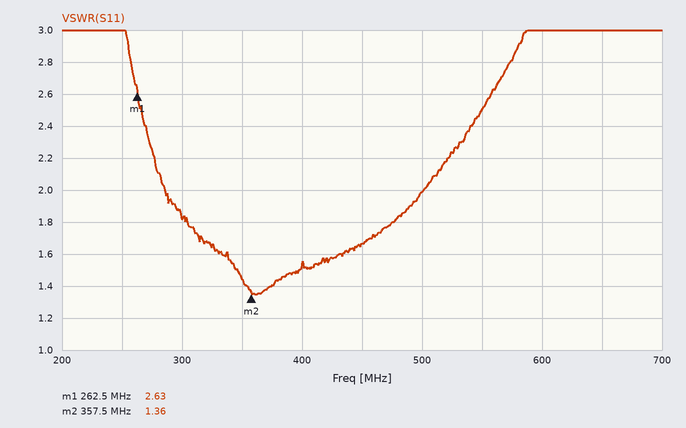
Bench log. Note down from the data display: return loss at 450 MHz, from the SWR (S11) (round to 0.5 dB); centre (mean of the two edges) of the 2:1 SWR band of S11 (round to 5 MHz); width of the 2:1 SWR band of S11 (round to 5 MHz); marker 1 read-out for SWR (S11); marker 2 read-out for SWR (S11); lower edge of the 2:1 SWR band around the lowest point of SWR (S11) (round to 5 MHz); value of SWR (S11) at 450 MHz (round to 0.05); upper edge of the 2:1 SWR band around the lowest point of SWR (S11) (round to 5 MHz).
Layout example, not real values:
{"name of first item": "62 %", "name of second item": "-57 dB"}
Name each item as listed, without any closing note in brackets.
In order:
{"return loss at 450 MHz, from the SWR (S11)": "12.0 dB", "centre (mean of the two edges) of the 2:1 SWR band of S11": "395 MHz", "width of the 2:1 SWR band of S11": "215 MHz", "marker 1 read-out for SWR": "2.63", "marker 2 read-out for SWR": "1.36", "lower edge of the 2:1 SWR band around the lowest point of SWR (S11)": "285 MHz", "value of SWR (S11) at 450 MHz": "1.65", "upper edge of the 2:1 SWR band around the lowest point of SWR (S11)": "500 MHz"}
